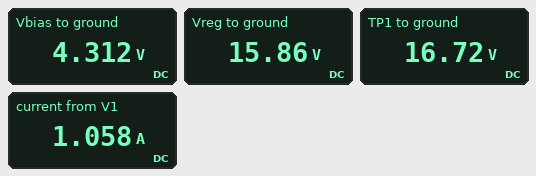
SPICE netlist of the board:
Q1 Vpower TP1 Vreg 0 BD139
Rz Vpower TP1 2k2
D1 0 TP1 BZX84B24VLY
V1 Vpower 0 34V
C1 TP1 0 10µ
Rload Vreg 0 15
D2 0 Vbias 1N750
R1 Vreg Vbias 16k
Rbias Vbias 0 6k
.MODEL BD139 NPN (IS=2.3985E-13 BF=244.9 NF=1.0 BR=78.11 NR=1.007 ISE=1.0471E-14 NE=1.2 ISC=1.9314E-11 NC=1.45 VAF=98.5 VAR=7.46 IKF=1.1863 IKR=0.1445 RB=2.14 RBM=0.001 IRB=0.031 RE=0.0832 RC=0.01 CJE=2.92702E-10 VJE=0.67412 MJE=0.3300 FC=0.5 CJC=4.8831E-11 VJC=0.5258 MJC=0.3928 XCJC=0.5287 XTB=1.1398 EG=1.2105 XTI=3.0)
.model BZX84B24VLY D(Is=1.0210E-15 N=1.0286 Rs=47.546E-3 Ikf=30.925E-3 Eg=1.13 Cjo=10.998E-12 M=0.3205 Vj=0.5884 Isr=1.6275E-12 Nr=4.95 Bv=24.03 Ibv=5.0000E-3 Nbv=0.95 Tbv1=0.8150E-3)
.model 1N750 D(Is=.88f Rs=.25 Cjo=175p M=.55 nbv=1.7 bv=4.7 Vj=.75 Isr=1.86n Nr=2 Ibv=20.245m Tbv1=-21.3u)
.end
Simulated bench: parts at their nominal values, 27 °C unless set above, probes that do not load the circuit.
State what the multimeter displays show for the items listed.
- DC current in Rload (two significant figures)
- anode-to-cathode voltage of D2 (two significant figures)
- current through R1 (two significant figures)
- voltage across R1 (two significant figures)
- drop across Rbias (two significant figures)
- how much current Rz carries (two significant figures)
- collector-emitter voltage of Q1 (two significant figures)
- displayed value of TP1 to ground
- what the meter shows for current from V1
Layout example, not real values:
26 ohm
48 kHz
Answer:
1.1 A
-4.3 V
720 µA
12 V
4.3 V
7.9 mA
18 V
16.72 V
1.058 A
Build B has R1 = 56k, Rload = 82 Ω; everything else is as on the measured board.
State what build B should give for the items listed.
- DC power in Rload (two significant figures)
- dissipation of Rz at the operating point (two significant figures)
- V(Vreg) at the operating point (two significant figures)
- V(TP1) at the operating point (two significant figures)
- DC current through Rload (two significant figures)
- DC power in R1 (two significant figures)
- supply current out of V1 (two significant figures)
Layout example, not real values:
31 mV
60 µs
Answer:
6.6 W
45 mW
23 V
24 V
280 mA
7.9 mW
290 mA
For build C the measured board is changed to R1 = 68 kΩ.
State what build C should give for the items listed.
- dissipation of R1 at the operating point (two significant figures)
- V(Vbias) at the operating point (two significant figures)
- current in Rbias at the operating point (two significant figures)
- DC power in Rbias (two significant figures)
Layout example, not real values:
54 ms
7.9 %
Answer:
3.1 mW
1.3 V
210 µA
280 µW
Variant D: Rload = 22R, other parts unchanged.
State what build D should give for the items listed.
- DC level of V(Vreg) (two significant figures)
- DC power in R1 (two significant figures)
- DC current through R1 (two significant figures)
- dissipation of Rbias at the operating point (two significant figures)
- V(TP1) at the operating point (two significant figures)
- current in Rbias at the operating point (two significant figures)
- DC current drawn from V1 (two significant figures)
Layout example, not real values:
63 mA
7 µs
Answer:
19 V
14 mW
920 µA
3.4 mW
20 V
750 µA
880 mA
